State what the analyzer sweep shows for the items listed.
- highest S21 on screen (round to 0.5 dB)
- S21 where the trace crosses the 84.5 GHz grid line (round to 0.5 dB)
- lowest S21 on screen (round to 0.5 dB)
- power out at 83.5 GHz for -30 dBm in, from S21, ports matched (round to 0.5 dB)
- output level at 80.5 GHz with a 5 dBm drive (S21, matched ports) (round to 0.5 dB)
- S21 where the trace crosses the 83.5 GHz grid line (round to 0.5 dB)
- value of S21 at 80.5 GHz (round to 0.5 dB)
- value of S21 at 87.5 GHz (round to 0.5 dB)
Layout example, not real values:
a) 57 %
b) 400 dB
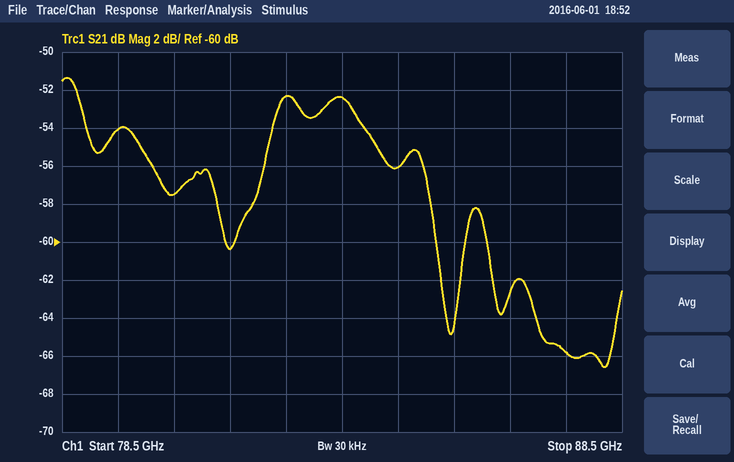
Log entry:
a) -51.5 dB
b) -56.0 dB
c) -66.5 dB
d) -82.5 dBm
e) -52.5 dBm
f) -52.5 dB
g) -57.5 dB
h) -66.0 dB
